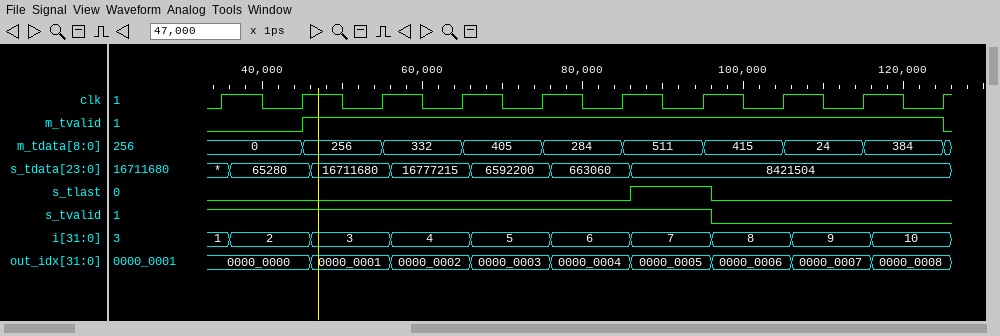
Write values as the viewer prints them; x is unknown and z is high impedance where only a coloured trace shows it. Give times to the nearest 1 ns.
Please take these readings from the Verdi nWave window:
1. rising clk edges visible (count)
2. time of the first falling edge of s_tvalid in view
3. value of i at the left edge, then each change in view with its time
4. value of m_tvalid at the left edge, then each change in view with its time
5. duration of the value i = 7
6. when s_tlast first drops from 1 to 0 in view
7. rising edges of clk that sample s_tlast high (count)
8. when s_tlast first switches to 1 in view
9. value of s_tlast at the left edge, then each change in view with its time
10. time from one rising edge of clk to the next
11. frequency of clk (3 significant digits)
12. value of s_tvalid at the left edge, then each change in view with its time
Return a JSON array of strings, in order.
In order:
["10", "96 ns", "1, 2 at 36 ns, 3 at 46 ns, 4 at 56 ns, 5 at 66 ns, 6 at 76 ns, 7 at 86 ns, 8 at 96 ns, 9 at 106 ns, 10 at 116 ns", "0, 1 at 45 ns, 0 at 125 ns", "10 ns", "96 ns", "1", "86 ns", "0, 1 at 86 ns, 0 at 96 ns", "10 ns", "100 MHz", "1, 0 at 96 ns"]
